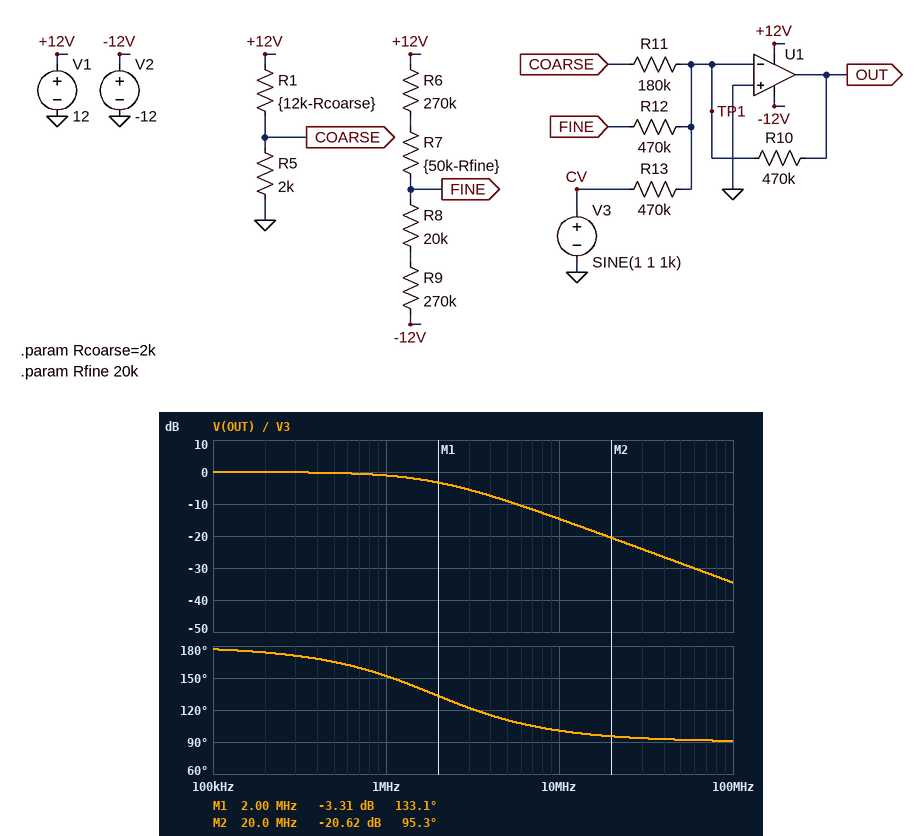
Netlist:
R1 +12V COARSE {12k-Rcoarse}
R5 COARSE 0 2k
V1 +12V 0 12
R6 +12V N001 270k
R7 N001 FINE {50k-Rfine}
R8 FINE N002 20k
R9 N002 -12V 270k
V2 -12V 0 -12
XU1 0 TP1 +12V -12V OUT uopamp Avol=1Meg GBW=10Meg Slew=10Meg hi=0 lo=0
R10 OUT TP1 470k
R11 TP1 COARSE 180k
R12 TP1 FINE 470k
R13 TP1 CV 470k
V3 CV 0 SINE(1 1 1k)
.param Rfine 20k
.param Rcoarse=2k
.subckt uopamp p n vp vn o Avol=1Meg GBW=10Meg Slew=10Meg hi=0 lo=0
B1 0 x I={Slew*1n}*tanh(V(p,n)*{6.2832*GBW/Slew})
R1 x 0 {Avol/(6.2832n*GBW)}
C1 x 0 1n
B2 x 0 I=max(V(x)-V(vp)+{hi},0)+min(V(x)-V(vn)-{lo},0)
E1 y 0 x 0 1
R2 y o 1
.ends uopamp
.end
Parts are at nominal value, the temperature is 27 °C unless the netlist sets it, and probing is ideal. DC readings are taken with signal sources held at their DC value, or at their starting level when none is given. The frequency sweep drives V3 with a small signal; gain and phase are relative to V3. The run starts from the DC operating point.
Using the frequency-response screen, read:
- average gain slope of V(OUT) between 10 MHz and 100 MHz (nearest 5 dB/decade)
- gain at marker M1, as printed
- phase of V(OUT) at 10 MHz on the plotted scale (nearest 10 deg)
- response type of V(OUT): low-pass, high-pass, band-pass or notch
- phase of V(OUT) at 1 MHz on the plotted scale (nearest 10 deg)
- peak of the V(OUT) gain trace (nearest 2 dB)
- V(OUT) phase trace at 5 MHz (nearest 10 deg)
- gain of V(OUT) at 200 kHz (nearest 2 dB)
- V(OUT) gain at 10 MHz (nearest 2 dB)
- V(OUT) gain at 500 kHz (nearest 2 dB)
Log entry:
-20 dB/decade
-3.31 dB
100 deg
low-pass
150 deg
0 dB
110 deg
0 dB
-14 dB
0 dB
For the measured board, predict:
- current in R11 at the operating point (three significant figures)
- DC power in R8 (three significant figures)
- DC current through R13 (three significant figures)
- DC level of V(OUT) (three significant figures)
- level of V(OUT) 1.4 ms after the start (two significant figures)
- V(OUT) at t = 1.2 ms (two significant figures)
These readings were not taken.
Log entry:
11.0 µA
33.4 µW
2.13 µA
-6.02 V
-6.6 V
-7.0 V
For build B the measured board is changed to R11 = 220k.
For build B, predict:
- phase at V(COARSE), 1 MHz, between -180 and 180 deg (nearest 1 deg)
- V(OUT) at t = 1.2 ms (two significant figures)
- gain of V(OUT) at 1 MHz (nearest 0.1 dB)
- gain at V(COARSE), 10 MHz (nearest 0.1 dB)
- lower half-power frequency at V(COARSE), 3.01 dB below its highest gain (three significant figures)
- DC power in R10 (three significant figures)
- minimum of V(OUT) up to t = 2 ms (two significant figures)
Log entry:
64 deg
-6.0 V
-0.9 dB
-56.4 dB
2.05 MHz
55.0 µW
-6.1 V
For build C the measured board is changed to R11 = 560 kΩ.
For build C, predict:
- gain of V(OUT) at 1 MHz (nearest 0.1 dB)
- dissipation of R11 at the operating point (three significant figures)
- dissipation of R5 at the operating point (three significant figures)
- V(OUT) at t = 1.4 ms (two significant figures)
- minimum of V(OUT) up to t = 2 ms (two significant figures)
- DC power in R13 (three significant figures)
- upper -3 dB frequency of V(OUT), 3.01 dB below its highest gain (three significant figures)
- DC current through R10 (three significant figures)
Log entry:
-0.5 dB
7.10 µW
1.99 mW
-3.1 V
-3.5 V
2.13 µW
2.78 MHz
5.36 µA
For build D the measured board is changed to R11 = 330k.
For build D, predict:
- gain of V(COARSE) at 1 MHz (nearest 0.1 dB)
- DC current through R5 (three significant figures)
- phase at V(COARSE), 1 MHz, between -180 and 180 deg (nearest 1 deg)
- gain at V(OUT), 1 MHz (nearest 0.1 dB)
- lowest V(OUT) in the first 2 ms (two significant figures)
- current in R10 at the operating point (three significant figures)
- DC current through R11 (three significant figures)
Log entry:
-66.7 dB
995 µA
67 deg
-0.7 dB
-4.7 V
7.83 µA
6.03 µA
